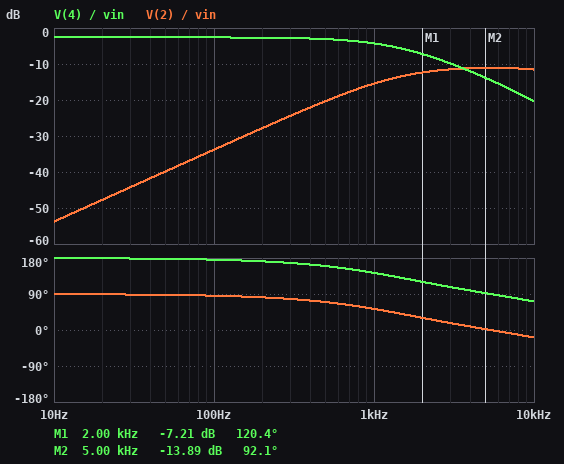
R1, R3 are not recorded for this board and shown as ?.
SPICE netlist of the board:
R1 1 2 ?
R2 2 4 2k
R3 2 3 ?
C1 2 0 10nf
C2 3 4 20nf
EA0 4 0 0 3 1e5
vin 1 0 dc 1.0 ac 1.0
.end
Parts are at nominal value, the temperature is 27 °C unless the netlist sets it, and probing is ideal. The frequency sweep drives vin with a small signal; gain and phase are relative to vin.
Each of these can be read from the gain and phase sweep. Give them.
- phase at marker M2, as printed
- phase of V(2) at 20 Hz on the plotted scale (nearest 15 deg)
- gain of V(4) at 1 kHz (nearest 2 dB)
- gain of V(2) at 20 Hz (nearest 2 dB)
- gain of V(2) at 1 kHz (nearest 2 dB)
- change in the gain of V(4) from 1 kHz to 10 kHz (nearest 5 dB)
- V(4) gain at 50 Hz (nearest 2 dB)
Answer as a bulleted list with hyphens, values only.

- 92.1 deg
- 90 deg
- -4 dB
- -48 dB
- -16 dB
- -15 dB
- -2 dB
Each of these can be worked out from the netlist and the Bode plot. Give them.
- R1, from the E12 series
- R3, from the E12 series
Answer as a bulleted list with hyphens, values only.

- 2.7 kΩ
- 2.2 kΩ
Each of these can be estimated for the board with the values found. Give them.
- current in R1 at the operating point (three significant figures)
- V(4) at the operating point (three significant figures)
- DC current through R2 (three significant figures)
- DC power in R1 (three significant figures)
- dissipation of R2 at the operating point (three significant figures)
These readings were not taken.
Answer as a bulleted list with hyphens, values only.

- 370 µA
- -741 mV
- 370 µA
- 370 µW
- 274 µW
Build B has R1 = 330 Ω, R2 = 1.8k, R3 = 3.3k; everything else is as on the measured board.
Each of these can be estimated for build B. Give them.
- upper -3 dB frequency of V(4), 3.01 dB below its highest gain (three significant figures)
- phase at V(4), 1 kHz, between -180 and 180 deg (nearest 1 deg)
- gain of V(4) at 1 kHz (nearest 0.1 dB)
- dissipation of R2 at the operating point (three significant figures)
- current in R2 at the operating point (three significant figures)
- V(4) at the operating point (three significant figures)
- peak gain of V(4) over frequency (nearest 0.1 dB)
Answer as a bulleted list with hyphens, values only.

- 346 Hz
- 108 deg
- 5.0 dB
- 16.5 mW
- 3.03 mA
- -5.45 V
- 14.7 dB
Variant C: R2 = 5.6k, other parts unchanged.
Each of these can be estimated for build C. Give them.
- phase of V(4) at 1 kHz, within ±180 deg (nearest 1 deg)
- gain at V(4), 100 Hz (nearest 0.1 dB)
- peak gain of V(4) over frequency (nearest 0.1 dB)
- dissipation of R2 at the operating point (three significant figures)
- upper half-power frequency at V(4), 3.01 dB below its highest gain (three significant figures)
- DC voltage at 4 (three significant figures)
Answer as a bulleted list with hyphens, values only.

- 120 deg
- 6.2 dB
- 6.3 dB
- 768 µW
- 671 Hz
- -2.07 V
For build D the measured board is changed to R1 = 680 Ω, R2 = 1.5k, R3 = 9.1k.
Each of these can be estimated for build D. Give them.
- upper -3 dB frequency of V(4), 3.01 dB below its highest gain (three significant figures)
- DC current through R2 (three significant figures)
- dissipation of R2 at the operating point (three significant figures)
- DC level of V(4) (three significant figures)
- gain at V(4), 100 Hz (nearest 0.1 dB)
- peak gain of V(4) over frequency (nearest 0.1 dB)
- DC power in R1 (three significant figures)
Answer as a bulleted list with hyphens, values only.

- 261 Hz
- 1.47 mA
- 3.24 mW
- -2.21 V
- 6.3 dB
- 6.9 dB
- 1.47 mW
